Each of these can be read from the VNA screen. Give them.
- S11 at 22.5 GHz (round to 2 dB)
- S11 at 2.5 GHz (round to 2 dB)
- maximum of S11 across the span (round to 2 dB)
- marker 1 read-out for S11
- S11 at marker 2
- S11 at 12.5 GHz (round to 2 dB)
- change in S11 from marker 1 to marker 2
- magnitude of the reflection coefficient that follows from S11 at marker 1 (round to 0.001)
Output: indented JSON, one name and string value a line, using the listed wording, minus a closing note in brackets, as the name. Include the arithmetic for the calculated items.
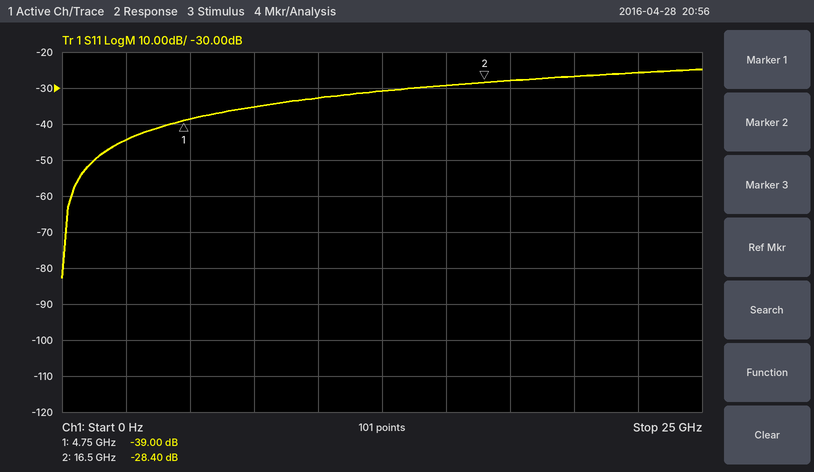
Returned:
{
  "S11 at 22.5 GHz": "-26 dB",
  "S11 at 2.5 GHz": "-44 dB",
  "maximum of S11 across the span": "-24 dB",
  "marker 1 read-out for S11": "-39.00 dB",
  "S11 at marker 2": "-28.40 dB",
  "S11 at 12.5 GHz": "-30 dB",
  "change in S11 from marker 1 to marker 2": "-28.4 − (-39) = 10.60 dB",
  "magnitude of the reflection coefficient that follows from S11 at marker 1": "10^(-39/20) ≈ 0.011"
}
